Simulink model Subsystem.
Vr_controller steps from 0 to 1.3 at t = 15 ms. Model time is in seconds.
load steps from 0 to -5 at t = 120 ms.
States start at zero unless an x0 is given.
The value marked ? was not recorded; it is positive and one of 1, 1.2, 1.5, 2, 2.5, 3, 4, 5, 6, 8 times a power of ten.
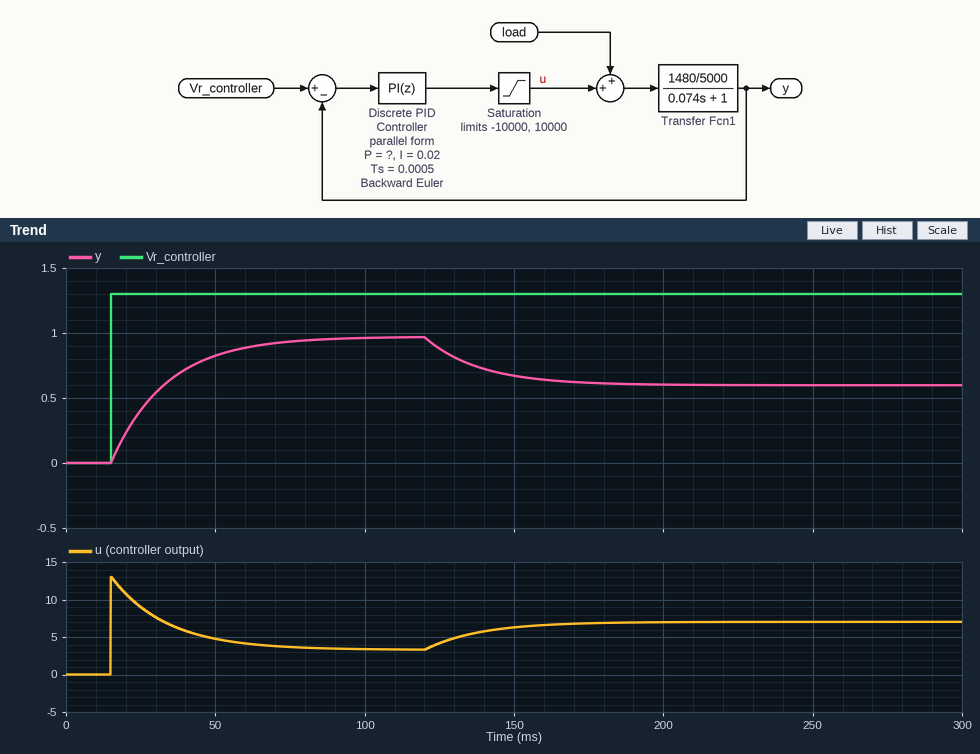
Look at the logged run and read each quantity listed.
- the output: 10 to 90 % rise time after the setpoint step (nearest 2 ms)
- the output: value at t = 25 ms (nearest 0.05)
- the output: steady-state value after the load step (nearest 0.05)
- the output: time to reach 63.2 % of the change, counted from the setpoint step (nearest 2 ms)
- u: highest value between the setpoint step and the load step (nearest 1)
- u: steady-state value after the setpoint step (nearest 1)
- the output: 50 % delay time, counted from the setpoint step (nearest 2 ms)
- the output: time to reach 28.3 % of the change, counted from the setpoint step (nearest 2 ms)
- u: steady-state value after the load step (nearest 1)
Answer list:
40 ms
0.40
0.60
18 ms
13
3
12 ms
6 ms
7
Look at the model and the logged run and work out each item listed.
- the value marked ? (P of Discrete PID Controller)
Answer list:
10
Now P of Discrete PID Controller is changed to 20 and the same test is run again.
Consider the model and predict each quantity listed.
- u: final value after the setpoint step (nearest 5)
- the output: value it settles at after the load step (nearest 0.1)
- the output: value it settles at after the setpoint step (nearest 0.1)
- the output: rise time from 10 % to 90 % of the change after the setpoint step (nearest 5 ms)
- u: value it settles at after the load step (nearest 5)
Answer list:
5
0.9
1.1
25 ms
10
